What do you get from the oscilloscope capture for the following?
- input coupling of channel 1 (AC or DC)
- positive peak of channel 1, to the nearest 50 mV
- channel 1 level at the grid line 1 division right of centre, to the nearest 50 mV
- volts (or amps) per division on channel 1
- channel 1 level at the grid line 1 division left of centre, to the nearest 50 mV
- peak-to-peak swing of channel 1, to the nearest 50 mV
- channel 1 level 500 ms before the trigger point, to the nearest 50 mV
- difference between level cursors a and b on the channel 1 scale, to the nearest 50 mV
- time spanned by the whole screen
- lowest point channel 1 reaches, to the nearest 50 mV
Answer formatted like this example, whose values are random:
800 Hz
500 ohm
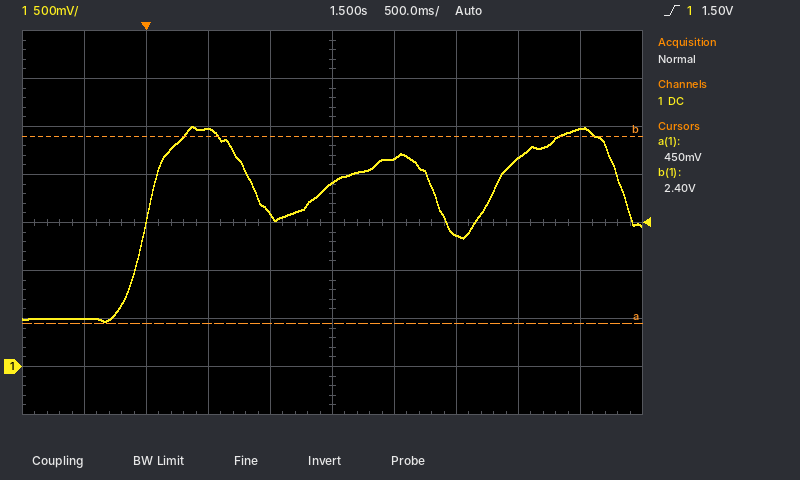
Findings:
DC
2.50 V
2.15 V
500 mV
1.60 V
2.05 V
500 mV
1.95 V
5 s
450 mV
